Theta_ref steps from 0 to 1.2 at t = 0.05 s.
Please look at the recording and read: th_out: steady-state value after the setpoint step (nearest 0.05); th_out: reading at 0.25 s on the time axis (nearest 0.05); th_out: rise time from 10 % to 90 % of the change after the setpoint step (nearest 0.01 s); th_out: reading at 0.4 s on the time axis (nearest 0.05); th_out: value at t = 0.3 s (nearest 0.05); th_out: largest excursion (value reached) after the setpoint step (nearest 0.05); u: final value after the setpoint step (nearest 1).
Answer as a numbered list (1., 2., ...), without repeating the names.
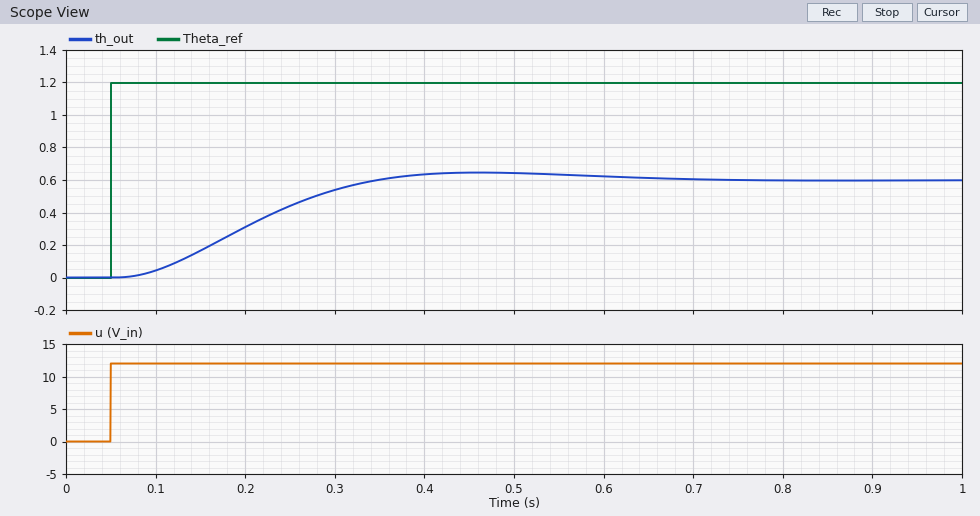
1. 0.60
2. 0.45
3. 0.19 s
4. 0.65
5. 0.55
6. 0.65
7. 12
